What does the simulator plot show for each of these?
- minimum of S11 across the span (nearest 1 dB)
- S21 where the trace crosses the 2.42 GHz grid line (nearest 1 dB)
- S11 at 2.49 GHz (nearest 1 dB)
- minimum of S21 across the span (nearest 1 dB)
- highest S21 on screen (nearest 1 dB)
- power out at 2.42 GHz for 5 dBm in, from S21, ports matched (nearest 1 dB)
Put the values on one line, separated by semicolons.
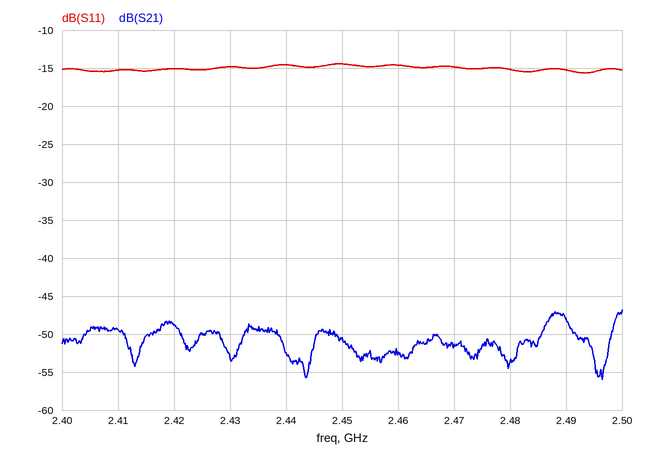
-16 dB; -49 dB; -15 dB; -56 dB; -47 dB; -44 dBm
